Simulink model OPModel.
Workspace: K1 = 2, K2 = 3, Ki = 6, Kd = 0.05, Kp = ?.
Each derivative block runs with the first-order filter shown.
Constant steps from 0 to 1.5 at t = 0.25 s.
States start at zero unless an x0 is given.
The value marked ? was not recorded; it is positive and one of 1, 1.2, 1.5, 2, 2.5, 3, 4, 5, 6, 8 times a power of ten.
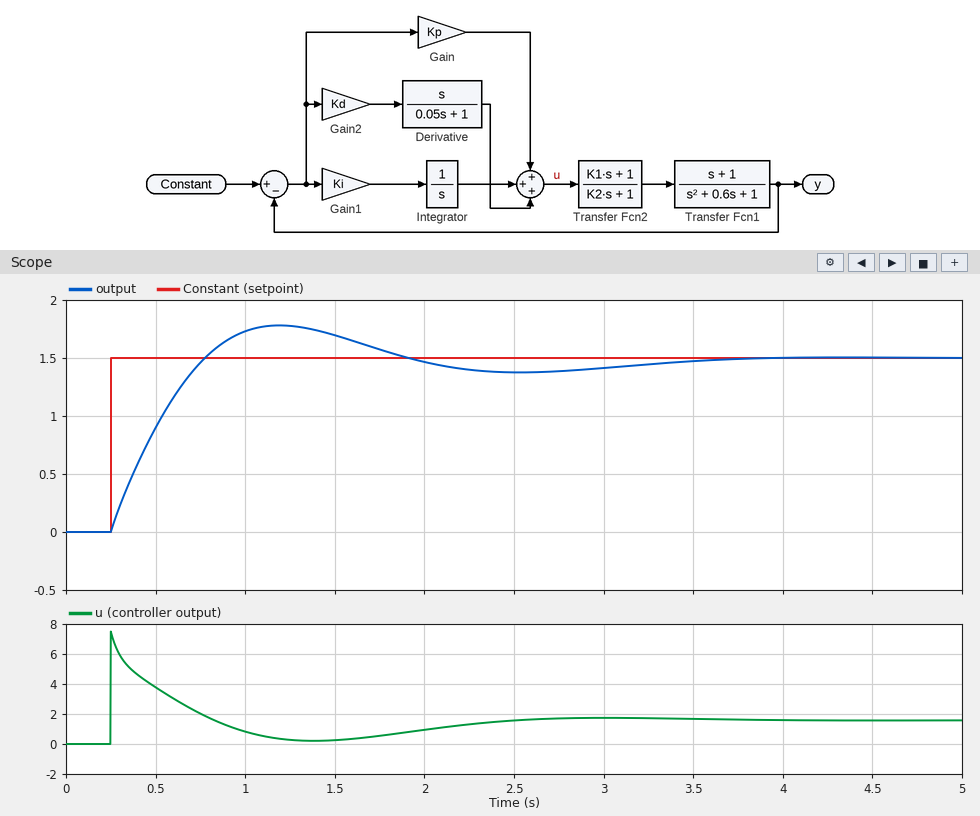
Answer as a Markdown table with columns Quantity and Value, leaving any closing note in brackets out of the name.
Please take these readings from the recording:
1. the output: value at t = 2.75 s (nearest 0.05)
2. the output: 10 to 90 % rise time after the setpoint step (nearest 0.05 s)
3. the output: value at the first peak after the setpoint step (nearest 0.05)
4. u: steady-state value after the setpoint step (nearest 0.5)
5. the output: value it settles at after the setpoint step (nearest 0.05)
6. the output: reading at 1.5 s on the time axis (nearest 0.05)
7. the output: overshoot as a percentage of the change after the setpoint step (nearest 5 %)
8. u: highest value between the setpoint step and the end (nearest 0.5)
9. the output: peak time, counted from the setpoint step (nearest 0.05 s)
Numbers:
| Quantity | Value |
|---|---|
| the output: value at t = 2.75 s | 1.40 |
| the output: 10 to 90 % rise time after the setpoint step | 0.40 s |
| the output: value at the first peak after the setpoint step | 1.80 |
| u: steady-state value after the setpoint step | 1.5 |
| the output: value it settles at after the setpoint step | 1.50 |
| the output: reading at 1.5 s on the time axis | 1.70 |
| the output: overshoot as a percentage of the change after the setpoint step | 20 % |
| u: highest value between the setpoint step and the end | 7.5 |
| the output: peak time, counted from the setpoint step | 0.95 s |
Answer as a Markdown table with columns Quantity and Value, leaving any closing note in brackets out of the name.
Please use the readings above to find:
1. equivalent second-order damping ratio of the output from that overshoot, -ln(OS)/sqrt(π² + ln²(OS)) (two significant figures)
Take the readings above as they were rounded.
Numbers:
| Quantity | Value |
|---|---|
| equivalent second-order damping ratio of the output from that overshoot, -ln(OS)/sqrt(π² + ln²(OS)) | 0.46 |
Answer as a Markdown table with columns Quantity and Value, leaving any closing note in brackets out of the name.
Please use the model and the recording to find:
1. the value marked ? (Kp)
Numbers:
| Quantity | Value |
|---|---|
| the value marked ? | 4 |
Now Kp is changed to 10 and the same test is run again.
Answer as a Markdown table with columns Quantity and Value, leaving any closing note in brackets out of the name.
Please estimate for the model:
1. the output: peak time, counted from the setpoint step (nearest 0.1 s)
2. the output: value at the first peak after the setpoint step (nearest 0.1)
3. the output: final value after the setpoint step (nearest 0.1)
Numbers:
| Quantity | Value |
|---|---|
| the output: peak time, counted from the setpoint step | 0.6 s |
| the output: value at the first peak after the setpoint step | 1.6 |
| the output: final value after the setpoint step | 1.5 |
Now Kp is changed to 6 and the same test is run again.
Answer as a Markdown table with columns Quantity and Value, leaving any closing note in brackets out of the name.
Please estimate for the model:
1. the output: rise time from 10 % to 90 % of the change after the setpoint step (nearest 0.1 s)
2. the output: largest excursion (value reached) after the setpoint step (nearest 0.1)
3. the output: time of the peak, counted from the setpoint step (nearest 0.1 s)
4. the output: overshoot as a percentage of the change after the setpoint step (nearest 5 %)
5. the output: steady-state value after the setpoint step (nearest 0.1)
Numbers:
| Quantity | Value |
|---|---|
| the output: rise time from 10 % to 90 % of the change after the setpoint step | 0.3 s |
| the output: largest excursion (value reached) after the setpoint step | 1.7 |
| the output: time of the peak, counted from the setpoint step | 0.8 s |
| the output: overshoot as a percentage of the change after the setpoint step | 10 % |
| the output: steady-state value after the setpoint step | 1.5 |
